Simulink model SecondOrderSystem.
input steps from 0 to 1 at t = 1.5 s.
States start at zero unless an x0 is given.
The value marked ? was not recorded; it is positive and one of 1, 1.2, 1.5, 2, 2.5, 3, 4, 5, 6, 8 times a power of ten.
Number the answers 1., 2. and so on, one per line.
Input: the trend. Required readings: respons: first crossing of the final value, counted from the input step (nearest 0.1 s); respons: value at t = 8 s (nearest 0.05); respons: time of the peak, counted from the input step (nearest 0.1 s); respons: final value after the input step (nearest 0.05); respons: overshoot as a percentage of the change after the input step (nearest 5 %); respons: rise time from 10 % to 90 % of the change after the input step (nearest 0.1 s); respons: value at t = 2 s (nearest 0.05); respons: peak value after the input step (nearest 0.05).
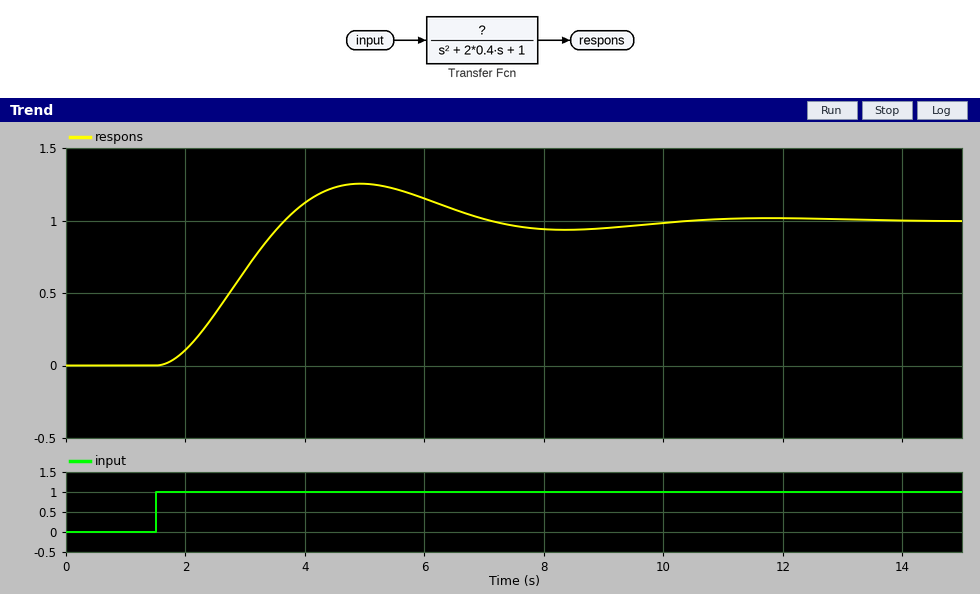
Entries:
1. 2.2 s
2. 0.95
3. 3.4 s
4. 1.00
5. 25 %
6. 1.5 s
7. 0.10
8. 1.25
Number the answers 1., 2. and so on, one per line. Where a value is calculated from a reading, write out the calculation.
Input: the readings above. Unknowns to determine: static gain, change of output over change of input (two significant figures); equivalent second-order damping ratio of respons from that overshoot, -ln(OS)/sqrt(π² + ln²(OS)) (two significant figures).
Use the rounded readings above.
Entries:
1. (1 - 0) / (1 - 0) = 1.0
2. ln(0.25) = -1.386; 1.386 / sqrt(9.870 + 1.922) = 0.40
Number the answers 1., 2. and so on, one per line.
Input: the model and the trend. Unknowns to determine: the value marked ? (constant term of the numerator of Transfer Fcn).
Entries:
1. 1
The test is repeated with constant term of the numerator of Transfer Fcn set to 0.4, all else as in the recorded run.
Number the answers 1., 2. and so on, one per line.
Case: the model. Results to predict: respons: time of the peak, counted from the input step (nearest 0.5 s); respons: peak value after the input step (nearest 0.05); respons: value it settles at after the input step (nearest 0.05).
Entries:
1. 3.5 s
2. 0.50
3. 0.40
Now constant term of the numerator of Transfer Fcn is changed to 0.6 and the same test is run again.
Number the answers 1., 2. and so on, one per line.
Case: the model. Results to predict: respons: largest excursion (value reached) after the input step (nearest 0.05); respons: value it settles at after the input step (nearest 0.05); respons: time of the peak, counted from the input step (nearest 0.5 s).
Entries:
1. 0.75
2. 0.60
3. 3.5 s
